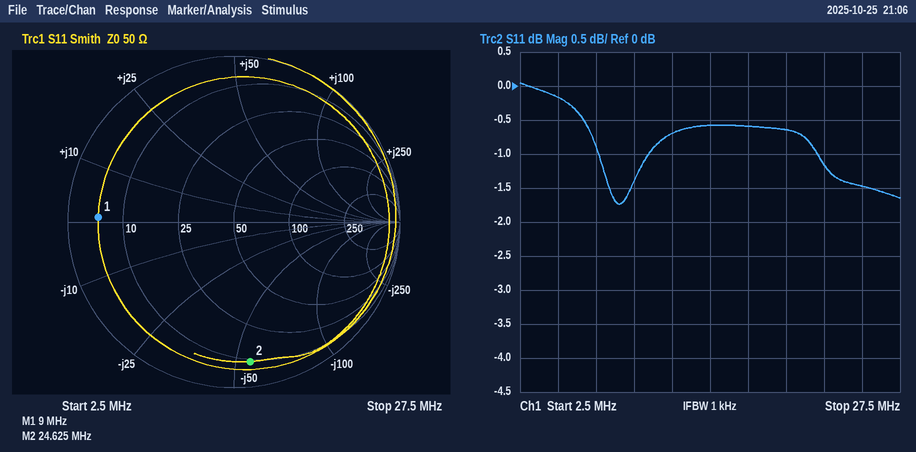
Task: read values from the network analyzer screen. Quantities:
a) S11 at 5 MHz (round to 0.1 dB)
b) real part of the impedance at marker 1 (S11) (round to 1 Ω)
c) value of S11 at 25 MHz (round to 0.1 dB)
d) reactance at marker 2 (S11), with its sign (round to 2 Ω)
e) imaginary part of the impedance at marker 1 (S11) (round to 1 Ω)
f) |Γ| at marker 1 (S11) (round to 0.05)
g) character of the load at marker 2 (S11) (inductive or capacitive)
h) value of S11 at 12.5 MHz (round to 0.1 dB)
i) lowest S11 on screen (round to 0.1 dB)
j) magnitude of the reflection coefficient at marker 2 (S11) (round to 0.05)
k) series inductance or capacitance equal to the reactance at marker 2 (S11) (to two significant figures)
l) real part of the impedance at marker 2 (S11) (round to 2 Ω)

-0.2 dB
5 Ω
-1.5 dB
-56 Ω
+1 Ω
0.80
capacitive
-0.7 dB
-1.7 dB
0.85
120 pF
10 Ω
